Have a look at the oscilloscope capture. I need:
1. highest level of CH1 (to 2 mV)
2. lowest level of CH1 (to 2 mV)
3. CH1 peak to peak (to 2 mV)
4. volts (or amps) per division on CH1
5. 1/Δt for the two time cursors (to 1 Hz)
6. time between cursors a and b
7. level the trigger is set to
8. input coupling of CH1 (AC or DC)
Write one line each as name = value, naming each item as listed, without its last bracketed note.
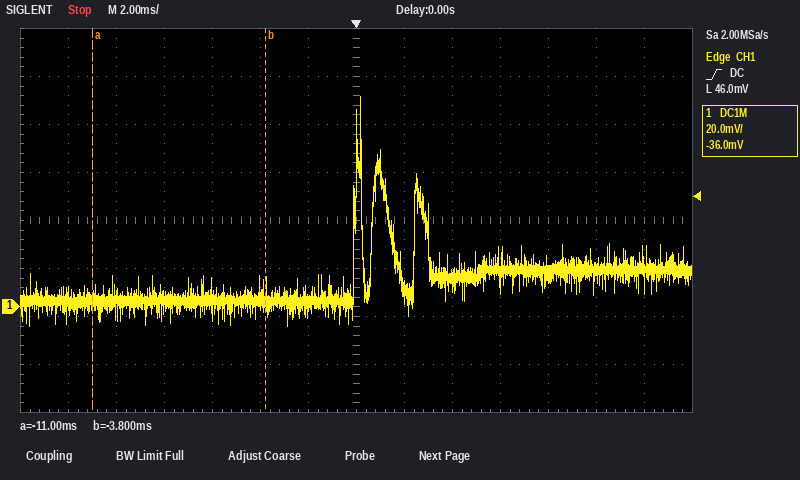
highest level of CH1 = 88 mV
lowest level of CH1 = -8 mV
CH1 peak to peak = 96 mV
volts (or amps) per division on CH1 = 20 mV
1/Δt for the two time cursors = 139 Hz
time between cursors a and b = 7.2 ms
level the trigger is set to = 46.0 mV
input coupling of CH1 = DC
